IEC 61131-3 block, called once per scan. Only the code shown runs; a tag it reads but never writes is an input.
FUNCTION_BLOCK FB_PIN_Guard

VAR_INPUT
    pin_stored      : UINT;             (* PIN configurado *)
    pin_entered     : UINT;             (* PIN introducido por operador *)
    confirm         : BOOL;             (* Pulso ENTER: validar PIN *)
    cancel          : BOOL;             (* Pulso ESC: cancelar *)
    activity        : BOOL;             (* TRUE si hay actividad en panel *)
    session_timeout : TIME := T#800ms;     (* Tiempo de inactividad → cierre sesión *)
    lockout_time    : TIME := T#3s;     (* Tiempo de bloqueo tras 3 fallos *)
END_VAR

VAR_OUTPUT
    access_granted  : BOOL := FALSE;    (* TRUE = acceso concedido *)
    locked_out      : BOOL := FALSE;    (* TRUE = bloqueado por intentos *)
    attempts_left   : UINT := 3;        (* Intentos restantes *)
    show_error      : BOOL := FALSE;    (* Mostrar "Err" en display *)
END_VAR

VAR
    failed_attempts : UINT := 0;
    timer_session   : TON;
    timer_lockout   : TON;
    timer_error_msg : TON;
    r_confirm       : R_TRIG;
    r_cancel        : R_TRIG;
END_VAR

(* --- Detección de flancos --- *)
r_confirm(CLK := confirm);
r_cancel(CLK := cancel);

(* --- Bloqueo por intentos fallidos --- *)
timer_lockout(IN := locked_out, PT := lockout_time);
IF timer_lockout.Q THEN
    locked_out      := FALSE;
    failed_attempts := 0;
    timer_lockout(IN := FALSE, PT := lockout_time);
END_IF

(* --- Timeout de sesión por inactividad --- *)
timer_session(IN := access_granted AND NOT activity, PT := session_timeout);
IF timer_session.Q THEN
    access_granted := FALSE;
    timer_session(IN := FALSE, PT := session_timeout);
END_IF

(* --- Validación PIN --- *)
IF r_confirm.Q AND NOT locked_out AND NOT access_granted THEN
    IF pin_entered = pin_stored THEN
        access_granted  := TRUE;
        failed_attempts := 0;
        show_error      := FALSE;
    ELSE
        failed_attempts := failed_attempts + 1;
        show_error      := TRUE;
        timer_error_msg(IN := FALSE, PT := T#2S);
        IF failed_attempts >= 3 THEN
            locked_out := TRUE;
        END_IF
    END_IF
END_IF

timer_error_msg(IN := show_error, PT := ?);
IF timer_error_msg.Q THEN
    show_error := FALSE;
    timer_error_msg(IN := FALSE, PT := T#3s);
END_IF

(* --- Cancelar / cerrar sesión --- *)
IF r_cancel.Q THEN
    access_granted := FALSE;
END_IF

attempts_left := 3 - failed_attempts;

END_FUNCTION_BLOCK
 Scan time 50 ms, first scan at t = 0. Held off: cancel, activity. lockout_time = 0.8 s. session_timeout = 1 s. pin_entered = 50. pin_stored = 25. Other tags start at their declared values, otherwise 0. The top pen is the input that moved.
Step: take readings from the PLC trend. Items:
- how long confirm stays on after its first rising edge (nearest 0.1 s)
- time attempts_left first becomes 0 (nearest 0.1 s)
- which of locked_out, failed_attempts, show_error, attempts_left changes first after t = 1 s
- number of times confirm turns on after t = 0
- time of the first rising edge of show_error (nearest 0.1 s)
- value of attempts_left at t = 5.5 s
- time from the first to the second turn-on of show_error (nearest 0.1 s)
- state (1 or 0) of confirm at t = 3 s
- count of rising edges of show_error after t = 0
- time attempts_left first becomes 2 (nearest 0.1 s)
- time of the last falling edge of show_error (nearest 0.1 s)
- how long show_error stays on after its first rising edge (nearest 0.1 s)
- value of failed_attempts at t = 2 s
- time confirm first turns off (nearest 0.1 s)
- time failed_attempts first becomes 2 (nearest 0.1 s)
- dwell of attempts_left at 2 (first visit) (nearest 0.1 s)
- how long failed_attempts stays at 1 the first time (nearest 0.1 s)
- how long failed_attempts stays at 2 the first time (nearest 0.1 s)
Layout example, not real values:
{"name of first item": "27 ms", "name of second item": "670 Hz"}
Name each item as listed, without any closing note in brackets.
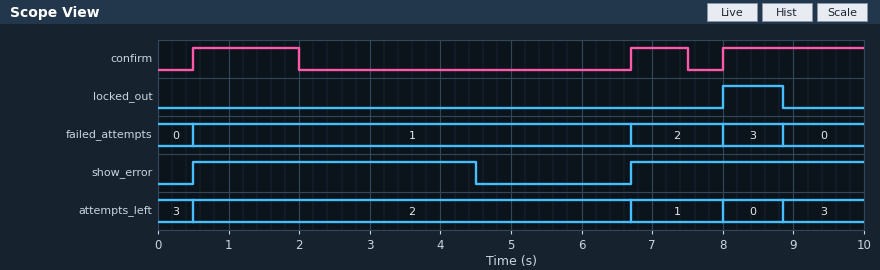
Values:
{"how long confirm stays on after its first rising edge": "1.5 s", "time attempts_left first becomes 0": "8.0 s", "which of locked_out, failed_attempts, show_error, attempts_left changes first after t = 1 s": "show_error", "number of times confirm turns on after t = 0": "3", "time of the first rising edge of show_error": "0.5 s", "value of attempts_left at t = 5.5 s": "2", "time from the first to the second turn-on of show_error": "6.2 s", "state (1 or 0) of confirm at t = 3 s": "0", "count of rising edges of show_error after t = 0": "2", "time attempts_left first becomes 2": "0.5 s", "time of the last falling edge of show_error": "4.5 s", "how long show_error stays on after its first rising edge": "4.0 s", "value of failed_attempts at t = 2 s": "1", "time confirm first turns off": "2.0 s", "time failed_attempts first becomes 2": "6.7 s", "dwell of attempts_left at 2 (first visit)": "6.2 s", "how long failed_attempts stays at 1 the first time": "6.2 s", "how long failed_attempts stays at 2 the first time": "1.3 s"}
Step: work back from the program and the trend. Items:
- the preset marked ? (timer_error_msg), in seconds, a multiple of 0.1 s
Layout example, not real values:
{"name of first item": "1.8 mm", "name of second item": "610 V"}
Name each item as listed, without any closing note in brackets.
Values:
{"the preset marked ? (timer_error_msg), in seconds, a multiple of 0.1 s": "4.0 s"}
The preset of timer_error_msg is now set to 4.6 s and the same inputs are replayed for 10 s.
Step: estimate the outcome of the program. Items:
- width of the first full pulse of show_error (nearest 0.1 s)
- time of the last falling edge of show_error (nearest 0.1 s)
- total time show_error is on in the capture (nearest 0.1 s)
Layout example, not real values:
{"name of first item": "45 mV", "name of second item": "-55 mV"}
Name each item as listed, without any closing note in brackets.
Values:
{"width of the first full pulse of show_error": "4.6 s", "time of the last falling edge of show_error": "5.1 s", "total time show_error is on in the capture": "7.9 s"}
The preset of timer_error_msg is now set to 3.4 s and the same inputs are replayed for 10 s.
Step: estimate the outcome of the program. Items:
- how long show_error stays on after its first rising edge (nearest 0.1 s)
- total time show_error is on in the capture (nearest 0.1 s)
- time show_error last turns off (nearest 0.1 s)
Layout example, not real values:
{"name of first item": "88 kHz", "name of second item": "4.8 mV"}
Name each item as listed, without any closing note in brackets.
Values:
{"how long show_error stays on after its first rising edge": "3.4 s", "total time show_error is on in the capture": "6.7 s", "time show_error last turns off": "3.9 s"}
